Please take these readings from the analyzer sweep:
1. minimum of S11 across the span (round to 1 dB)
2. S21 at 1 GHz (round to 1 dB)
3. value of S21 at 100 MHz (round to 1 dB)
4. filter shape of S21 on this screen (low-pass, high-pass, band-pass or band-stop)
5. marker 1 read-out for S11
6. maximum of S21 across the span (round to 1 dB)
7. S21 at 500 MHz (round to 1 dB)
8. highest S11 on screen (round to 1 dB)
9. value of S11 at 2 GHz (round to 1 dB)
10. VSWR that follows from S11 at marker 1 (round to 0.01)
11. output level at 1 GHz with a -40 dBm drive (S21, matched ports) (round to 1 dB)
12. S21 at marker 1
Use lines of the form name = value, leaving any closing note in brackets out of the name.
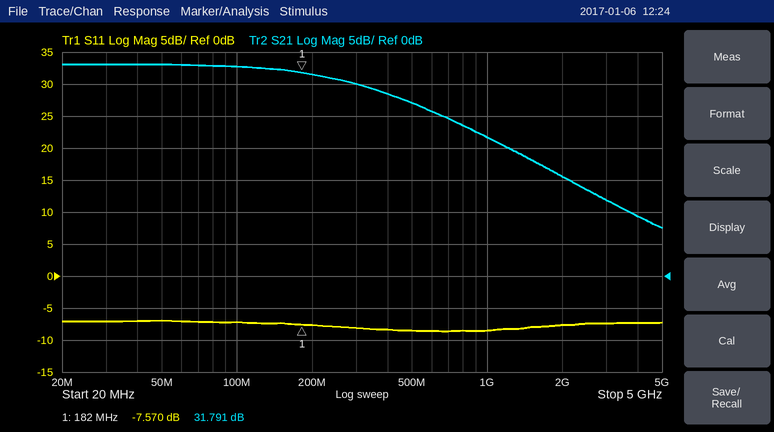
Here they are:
minimum of S11 across the span = -9 dB
S21 at 1 GHz = 22 dB
value of S21 at 100 MHz = 33 dB
filter shape of S21 on this screen = low-pass
marker 1 read-out for S11 = -7.570 dB
maximum of S21 across the span = 33 dB
S21 at 500 MHz = 27 dB
highest S11 on screen = -7 dB
value of S11 at 2 GHz = -8 dB
VSWR that follows from S11 at marker 1 = 2.44
output level at 1 GHz with a -40 dBm drive (S21, matched ports) = -18 dBm
S21 at marker 1 = 31.791 dB
